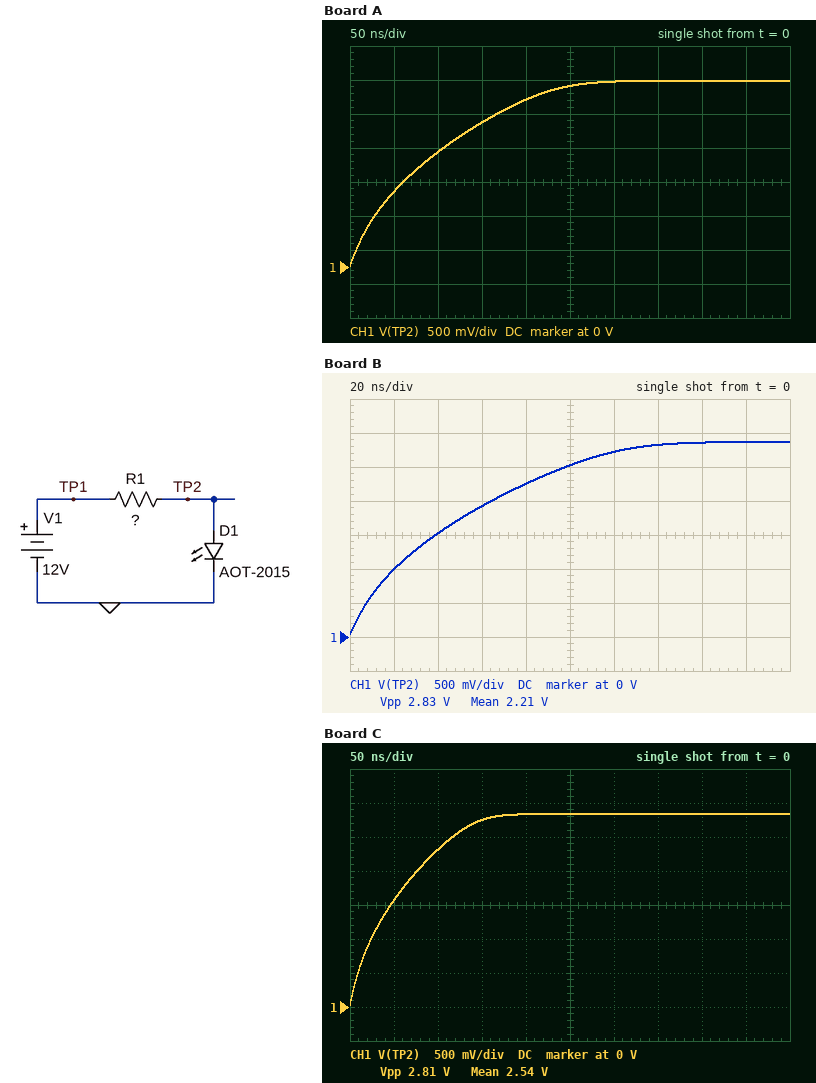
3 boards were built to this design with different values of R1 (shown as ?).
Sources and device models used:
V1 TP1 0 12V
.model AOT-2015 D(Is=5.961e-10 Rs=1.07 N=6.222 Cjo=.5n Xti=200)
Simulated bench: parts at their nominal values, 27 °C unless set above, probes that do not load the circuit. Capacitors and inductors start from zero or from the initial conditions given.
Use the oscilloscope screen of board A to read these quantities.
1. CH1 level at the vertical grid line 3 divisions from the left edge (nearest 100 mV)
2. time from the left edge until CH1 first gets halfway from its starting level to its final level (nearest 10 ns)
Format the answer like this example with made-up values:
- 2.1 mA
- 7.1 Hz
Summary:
- 2.1 V
- 70 ns
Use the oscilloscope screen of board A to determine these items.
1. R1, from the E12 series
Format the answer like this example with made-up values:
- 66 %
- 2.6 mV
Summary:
- 680 Ω
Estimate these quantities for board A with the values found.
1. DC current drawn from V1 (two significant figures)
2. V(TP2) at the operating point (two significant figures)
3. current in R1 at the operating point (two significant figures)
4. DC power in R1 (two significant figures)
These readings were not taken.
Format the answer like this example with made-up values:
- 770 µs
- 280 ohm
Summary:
- 14 mA
- 2.7 V
- 14 mA
- 130 mW
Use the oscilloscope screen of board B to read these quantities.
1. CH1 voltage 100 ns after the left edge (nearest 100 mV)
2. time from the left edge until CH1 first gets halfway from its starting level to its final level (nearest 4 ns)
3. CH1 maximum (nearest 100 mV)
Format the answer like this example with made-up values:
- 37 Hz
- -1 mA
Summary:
- 2.5 V
- 36 ns
- 2.9 V
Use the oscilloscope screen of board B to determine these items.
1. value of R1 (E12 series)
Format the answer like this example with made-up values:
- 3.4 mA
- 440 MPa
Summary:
- 330 Ω
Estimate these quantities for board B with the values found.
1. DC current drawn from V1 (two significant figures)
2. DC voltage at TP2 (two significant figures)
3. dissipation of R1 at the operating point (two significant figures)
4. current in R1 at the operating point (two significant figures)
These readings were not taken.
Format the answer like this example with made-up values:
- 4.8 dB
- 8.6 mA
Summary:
- 28 mA
- 2.9 V
- 250 mW
- 28 mA
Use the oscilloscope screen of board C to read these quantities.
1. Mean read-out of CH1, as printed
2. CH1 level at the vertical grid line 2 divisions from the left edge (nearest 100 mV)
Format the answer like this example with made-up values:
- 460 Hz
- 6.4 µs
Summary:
- 2.54 V
- 2.3 V
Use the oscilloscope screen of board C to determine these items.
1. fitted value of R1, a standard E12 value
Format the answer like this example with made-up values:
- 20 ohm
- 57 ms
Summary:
- 390 Ω
